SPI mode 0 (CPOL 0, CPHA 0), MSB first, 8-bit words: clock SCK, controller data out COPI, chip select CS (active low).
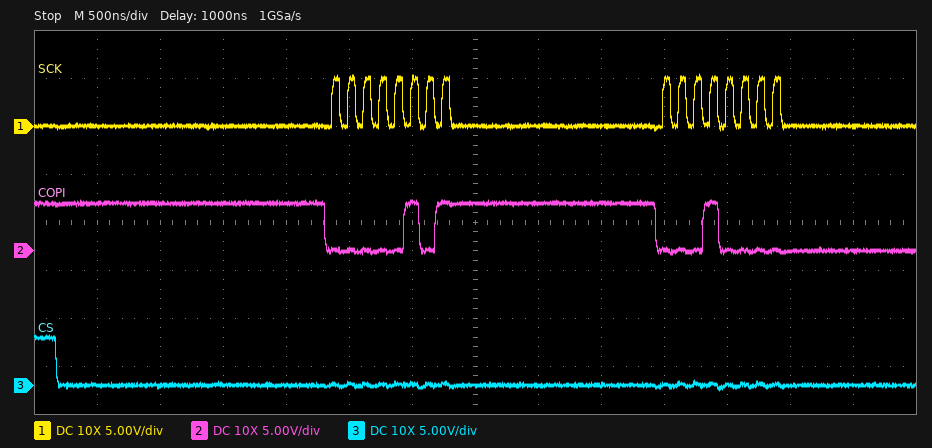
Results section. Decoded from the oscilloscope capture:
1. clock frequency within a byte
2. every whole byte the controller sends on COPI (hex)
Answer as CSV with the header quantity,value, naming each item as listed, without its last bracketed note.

quantity,value
clock frequency within a byte,8 MHz
every whole byte the controller sends on COPI,05 10
